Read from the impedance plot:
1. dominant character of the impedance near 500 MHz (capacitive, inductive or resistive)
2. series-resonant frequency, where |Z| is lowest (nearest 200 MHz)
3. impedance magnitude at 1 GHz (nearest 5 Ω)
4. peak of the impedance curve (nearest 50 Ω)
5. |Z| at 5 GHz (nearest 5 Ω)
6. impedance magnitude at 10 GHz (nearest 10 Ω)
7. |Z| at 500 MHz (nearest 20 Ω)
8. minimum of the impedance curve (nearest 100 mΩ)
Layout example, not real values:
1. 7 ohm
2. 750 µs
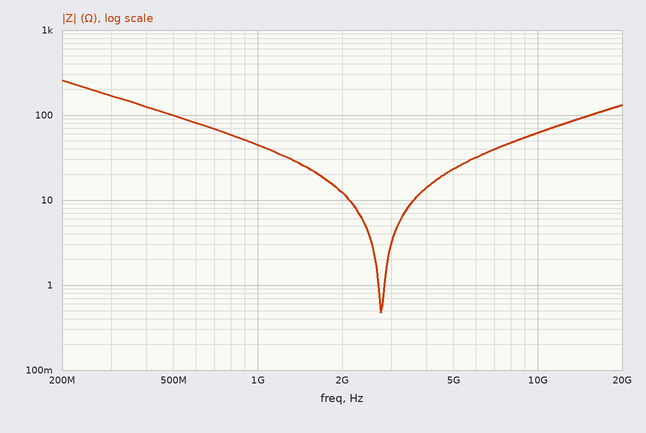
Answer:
1. capacitive
2. 2.8 GHz
3. 45 Ω
4. 250 Ω
5. 25 Ω
6. 60 Ω
7. 100 Ω
8. 500 mΩ
